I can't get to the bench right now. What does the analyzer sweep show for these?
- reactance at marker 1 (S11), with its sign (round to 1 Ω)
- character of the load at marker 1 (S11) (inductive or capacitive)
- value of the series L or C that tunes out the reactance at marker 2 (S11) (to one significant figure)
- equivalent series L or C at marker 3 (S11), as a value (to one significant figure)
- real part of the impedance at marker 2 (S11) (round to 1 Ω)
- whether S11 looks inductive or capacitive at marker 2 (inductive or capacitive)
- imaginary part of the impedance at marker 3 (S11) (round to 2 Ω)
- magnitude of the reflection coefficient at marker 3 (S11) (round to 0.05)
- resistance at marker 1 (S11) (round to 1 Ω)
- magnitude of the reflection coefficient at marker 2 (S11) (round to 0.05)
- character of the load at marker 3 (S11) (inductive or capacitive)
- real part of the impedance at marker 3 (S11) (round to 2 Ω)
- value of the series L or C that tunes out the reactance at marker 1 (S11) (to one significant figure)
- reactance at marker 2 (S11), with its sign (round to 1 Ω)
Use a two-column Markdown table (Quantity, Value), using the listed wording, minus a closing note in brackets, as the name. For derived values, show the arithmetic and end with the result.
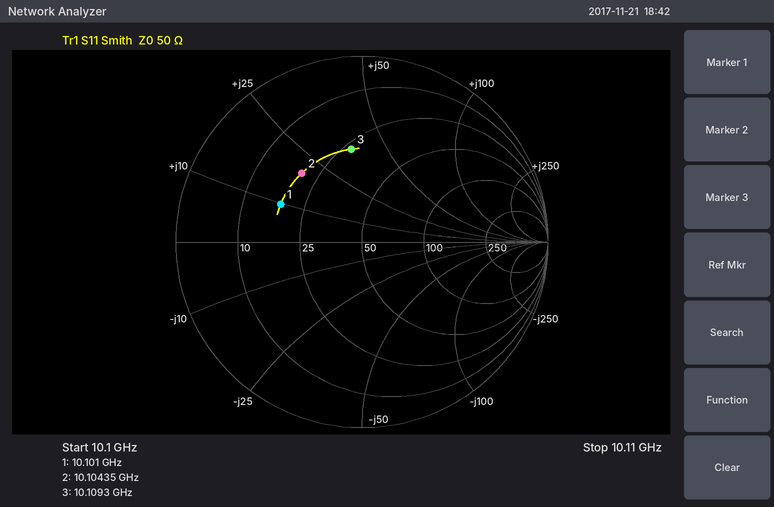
| Quantity | Value |
|---|---|
| reactance at marker 1 (S11), with its sign | +10 Ω |
| character of the load at marker 1 (S11) | inductive |
| value of the series L or C that tunes out the reactance at marker 2 (S11) | C = 1/(2π × 10.10435 GHz × 20 Ω) ≈ 788 fF, so 800 fF to one significant figure |
| equivalent series L or C at marker 3 (S11), as a value | L = 36 Ω/(2π × 10.1093 GHz) ≈ 567 pH, so 600 pH to one significant figure |
| real part of the impedance at marker 2 (S11) | 20 Ω |
| whether S11 looks inductive or capacitive at marker 2 | inductive |
| imaginary part of the impedance at marker 3 (S11) | +36 Ω |
| magnitude of the reflection coefficient at marker 3 (S11) | 0.50 |
| resistance at marker 1 (S11) | 18 Ω |
| magnitude of the reflection coefficient at marker 2 (S11) | 0.50 |
| character of the load at marker 3 (S11) | inductive |
| real part of the impedance at marker 3 (S11) | 28 Ω |
| value of the series L or C that tunes out the reactance at marker 1 (S11) | C = 1/(2π × 10.101 GHz × 10 Ω) ≈ 2 pF |
| reactance at marker 2 (S11), with its sign | +20 Ω |
